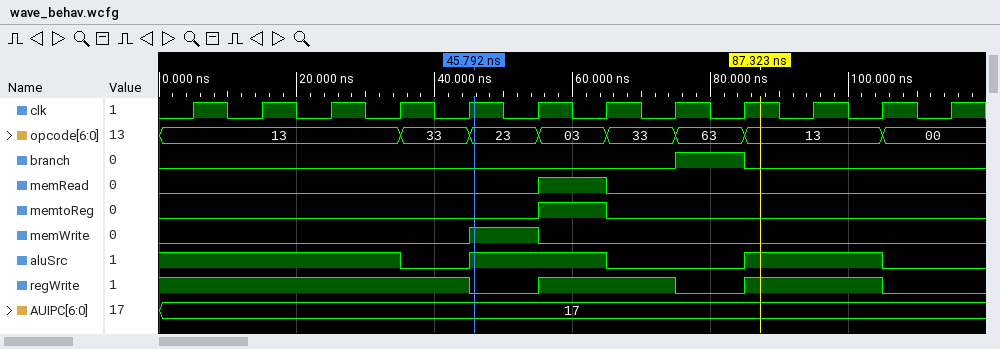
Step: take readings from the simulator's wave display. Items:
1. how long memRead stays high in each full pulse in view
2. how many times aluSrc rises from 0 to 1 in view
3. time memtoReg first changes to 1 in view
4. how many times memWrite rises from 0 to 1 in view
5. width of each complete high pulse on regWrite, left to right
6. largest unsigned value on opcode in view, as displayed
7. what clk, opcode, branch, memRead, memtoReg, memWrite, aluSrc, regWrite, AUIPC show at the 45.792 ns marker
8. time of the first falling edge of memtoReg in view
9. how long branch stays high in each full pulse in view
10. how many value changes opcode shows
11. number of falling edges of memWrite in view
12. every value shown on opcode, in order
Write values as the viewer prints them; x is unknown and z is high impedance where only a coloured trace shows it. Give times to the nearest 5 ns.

10 ns
2
55 ns
1
20 ns, 20 ns
63
clk=1, opcode=23, branch=0, memRead=0, memtoReg=0, memWrite=1, aluSrc=1, regWrite=0, AUIPC=17
65 ns
10 ns
7
1
13, 33, 23, 03, 33, 63, 13, 00
